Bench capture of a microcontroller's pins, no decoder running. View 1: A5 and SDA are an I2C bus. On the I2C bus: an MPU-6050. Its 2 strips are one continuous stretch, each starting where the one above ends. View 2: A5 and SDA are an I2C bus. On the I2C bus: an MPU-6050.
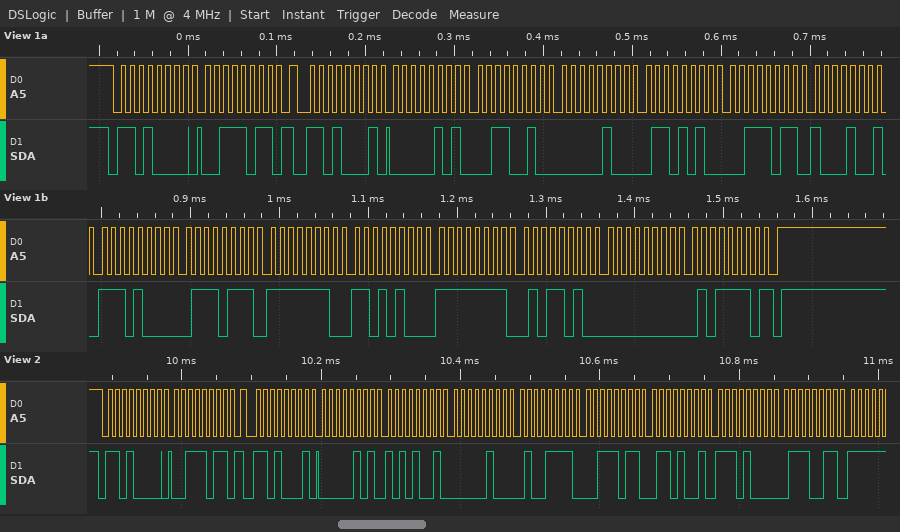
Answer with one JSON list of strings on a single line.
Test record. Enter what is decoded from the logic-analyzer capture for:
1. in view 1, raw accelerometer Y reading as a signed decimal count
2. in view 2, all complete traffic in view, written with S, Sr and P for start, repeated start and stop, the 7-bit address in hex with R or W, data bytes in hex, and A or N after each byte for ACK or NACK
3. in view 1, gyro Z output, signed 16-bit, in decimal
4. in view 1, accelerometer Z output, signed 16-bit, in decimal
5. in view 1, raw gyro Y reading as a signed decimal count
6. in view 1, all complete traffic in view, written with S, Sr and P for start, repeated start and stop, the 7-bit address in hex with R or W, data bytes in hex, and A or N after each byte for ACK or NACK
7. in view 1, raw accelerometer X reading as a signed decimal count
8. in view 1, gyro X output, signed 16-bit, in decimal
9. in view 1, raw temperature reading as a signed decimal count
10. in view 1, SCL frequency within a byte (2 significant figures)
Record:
["1130", "S 68W A 3B A Sr 68R A 05 A A9 A 04 A 4F A 3B A 69 A E8 A 73 A", "94", "15241", "-166", "S 68W A 3B A Sr 68R A 05 A 32 A 04 A 6A A 3B A 89 A E8 A 77 A FE A D4 A FF A 5A A 00 A 5E N P", "1330", "-300", "-6025", "100 kHz"]
